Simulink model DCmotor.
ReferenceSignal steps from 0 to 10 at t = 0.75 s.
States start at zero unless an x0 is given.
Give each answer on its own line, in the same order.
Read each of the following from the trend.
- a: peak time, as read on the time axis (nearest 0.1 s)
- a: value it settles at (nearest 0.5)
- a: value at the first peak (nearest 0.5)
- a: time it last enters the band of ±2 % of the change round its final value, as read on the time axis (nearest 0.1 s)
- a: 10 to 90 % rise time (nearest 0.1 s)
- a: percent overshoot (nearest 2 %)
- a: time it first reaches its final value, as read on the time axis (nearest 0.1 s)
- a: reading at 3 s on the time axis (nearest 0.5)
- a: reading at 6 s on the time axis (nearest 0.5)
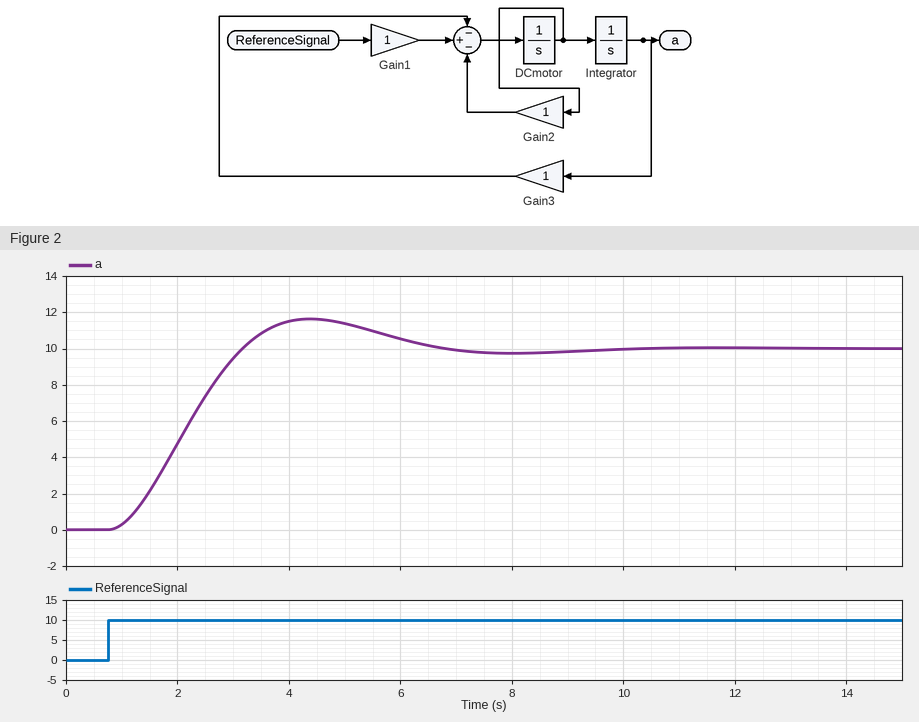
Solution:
4.4 s
10.0
11.5
8.8 s
1.6 s
16 %
3.2 s
9.5
10.5
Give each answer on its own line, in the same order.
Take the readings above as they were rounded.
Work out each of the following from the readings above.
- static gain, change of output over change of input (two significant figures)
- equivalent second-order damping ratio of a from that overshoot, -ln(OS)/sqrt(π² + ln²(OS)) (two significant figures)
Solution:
1.0
0.50
